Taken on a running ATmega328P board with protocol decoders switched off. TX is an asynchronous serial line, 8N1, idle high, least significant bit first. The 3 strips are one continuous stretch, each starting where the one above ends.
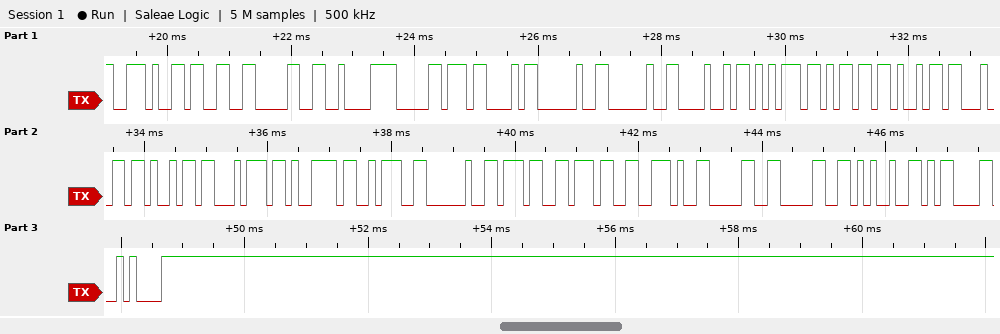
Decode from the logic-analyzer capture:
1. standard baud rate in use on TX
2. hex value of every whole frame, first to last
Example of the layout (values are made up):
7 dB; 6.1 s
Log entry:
9600 baud; 2E 33 30 C2 B0 43 20 20 48 75 6D 69 64 69 74 79 3A 20 37 37 2E 30 30 25 0D 0A
